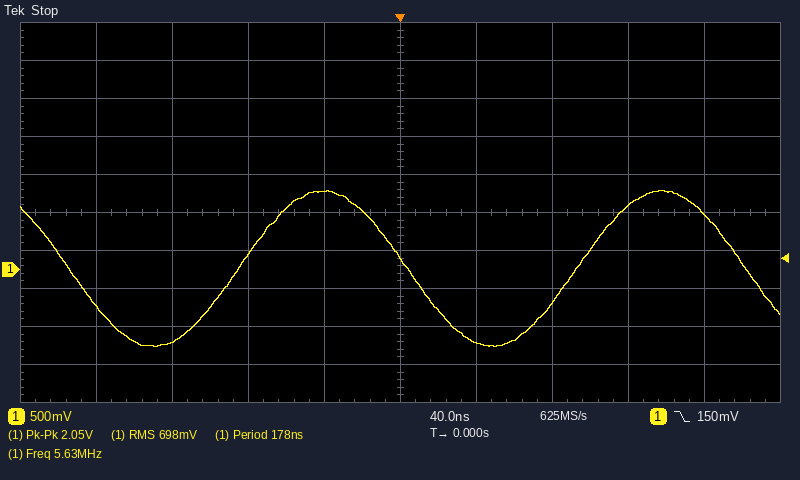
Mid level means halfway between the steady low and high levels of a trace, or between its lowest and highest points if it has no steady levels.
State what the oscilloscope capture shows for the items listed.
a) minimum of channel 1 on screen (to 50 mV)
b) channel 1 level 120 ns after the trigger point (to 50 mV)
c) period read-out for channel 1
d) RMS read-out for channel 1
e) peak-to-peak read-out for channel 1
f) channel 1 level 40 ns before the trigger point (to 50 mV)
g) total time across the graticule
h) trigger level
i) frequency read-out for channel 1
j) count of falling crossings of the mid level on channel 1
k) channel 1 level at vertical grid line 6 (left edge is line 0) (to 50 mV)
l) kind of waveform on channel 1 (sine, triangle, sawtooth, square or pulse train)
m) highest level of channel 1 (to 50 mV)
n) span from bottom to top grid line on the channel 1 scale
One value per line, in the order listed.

-1.00 V
850 mV
178 ns
698 mV
2.05 V
1.05 V
400 ns
150 mV
5.63 MHz
3
-950 mV
sine
1.05 V
5 V
